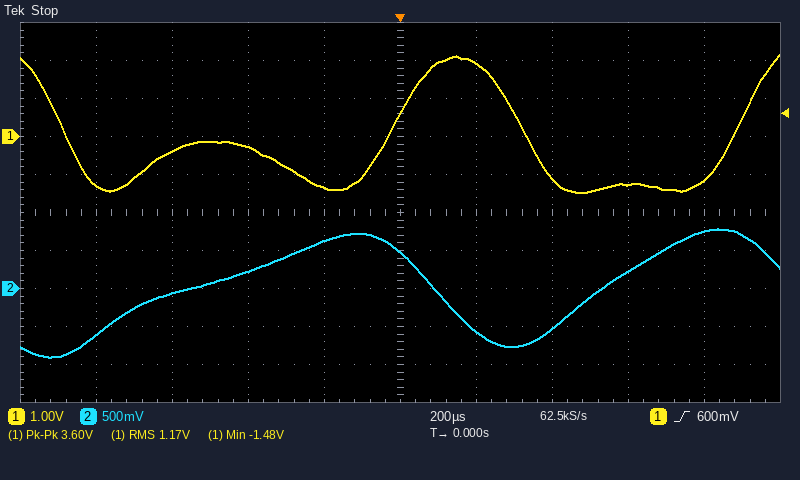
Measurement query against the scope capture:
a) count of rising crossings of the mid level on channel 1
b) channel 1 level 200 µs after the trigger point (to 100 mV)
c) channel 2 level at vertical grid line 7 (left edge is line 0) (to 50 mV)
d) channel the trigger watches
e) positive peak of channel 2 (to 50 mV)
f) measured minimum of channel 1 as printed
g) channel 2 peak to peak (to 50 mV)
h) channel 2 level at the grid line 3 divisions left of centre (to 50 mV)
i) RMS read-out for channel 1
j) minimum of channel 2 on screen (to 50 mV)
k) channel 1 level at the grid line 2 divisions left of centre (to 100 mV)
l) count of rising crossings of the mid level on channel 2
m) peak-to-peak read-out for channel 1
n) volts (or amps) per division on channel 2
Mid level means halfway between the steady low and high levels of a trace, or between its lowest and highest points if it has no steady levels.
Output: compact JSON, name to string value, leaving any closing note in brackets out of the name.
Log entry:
{"count of rising crossings of the mid level on channel 1": "2", "channel 1 level 200 µs after the trigger point": "1.9 V", "channel 2 level at vertical grid line 7 (left edge is line 0)": "-550 mV", "channel the trigger watches": "channel 1", "positive peak of channel 2": "800 mV", "measured minimum of channel 1 as printed": "-1.48 V", "channel 2 peak to peak": "1.70 V", "channel 2 level at the grid line 3 divisions left of centre": "-50 mV", "RMS read-out for channel 1": "1.17 V", "minimum of channel 2 on screen": "-900 mV", "channel 1 level at the grid line 2 divisions left of centre": "-300 mV", "count of rising crossings of the mid level on channel 2": "2", "peak-to-peak read-out for channel 1": "3.60 V", "volts (or amps) per division on channel 2": "500 mV"}
